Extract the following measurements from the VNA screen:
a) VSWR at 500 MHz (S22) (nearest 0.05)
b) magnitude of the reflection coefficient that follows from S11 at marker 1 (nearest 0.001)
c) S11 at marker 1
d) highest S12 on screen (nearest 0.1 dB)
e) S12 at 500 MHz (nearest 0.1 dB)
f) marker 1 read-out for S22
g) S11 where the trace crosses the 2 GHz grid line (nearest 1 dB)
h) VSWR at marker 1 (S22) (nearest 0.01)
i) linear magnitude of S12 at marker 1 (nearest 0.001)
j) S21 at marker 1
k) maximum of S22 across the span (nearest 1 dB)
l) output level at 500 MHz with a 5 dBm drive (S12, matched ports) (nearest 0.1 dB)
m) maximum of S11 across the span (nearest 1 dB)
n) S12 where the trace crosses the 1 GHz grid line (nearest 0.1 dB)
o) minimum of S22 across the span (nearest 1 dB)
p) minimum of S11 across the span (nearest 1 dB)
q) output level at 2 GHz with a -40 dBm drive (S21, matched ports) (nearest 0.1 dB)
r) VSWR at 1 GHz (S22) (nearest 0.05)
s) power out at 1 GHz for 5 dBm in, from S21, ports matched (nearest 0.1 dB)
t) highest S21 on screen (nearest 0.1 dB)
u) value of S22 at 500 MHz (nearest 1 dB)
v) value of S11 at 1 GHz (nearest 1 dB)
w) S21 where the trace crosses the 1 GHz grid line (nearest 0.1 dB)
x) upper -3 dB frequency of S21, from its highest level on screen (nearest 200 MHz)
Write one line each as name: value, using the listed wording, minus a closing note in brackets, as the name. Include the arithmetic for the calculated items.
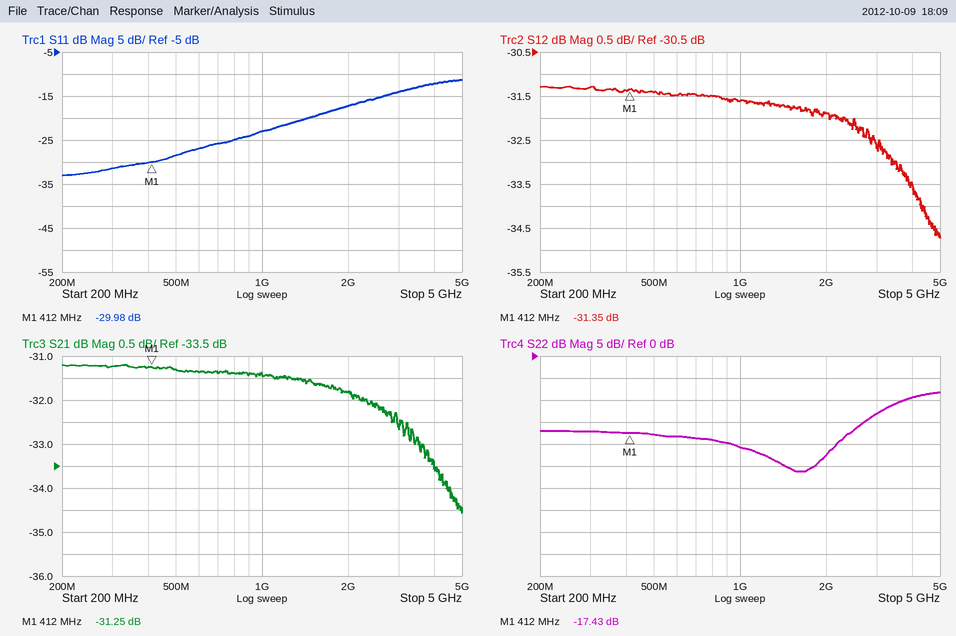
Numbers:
VSWR at 500 MHz (S22): |Γ| = 10^(-18/20) = 0.1259; VSWR = (1 + 0.1259)/(1 − 0.1259) ≈ 1.29, so 1.30 to the nearest 0.05
magnitude of the reflection coefficient that follows from S11 at marker 1: 10^(-29.98/20) ≈ 0.032
S11 at marker 1: -29.98 dB
highest S12 on screen: -31.3 dB
S12 at 500 MHz: -31.4 dB
marker 1 read-out for S22: -17.43 dB
S11 where the trace crosses the 2 GHz grid line: -17 dB
VSWR at marker 1 (S22): (1 + 0.1344)/(1 − 0.1344) ≈ 1.31
linear magnitude of S12 at marker 1: 10^(-31.35/20) ≈ 0.027
S21 at marker 1: -31.25 dB
maximum of S22 across the span: -8 dB
output level at 500 MHz with a 5 dBm drive (S12, matched ports): 5 dBm + (-31.4 dB) = -26.4 dBm
maximum of S11 across the span: -11 dB
S12 where the trace crosses the 1 GHz grid line: -31.6 dB
minimum of S22 across the span: -26 dB
minimum of S11 across the span: -33 dB
output level at 2 GHz with a -40 dBm drive (S21, matched ports): -40 dBm + (-31.8 dB) = -71.8 dBm
VSWR at 1 GHz (S22): |Γ| = 10^(-21/20) = 0.0891; VSWR = (1 + 0.0891)/(1 − 0.0891) ≈ 1.20
power out at 1 GHz for 5 dBm in, from S21, ports matched: 5 dBm + (-31.4 dB) = -26.4 dBm
highest S21 on screen: -31.2 dB
value of S22 at 500 MHz: -18 dB
value of S11 at 1 GHz: -23 dB
S21 where the trace crosses the 1 GHz grid line: -31.4 dB
upper -3 dB frequency of S21, from its highest level on screen: 4.6 GHz
